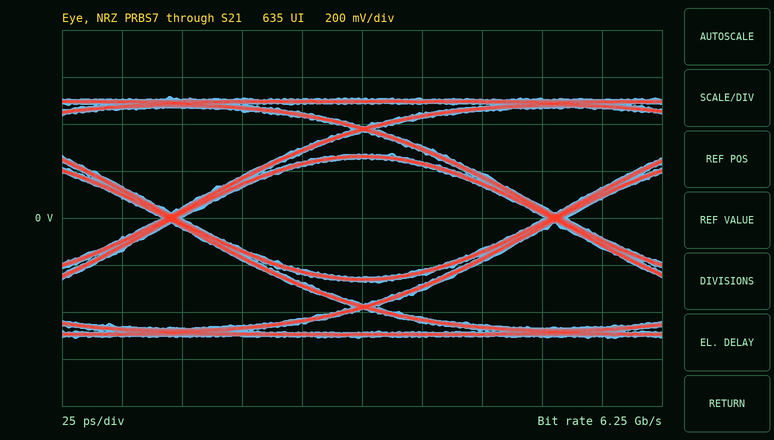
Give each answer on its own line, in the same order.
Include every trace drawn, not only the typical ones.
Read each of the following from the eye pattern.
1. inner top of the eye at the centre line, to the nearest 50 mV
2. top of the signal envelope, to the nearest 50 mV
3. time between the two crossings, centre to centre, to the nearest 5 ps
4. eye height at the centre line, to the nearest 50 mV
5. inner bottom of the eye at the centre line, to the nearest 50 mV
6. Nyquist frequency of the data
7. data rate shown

250 mV
500 mV
160 ps
500 mV
-250 mV
3.125 GHz
6.25 Gb/s
